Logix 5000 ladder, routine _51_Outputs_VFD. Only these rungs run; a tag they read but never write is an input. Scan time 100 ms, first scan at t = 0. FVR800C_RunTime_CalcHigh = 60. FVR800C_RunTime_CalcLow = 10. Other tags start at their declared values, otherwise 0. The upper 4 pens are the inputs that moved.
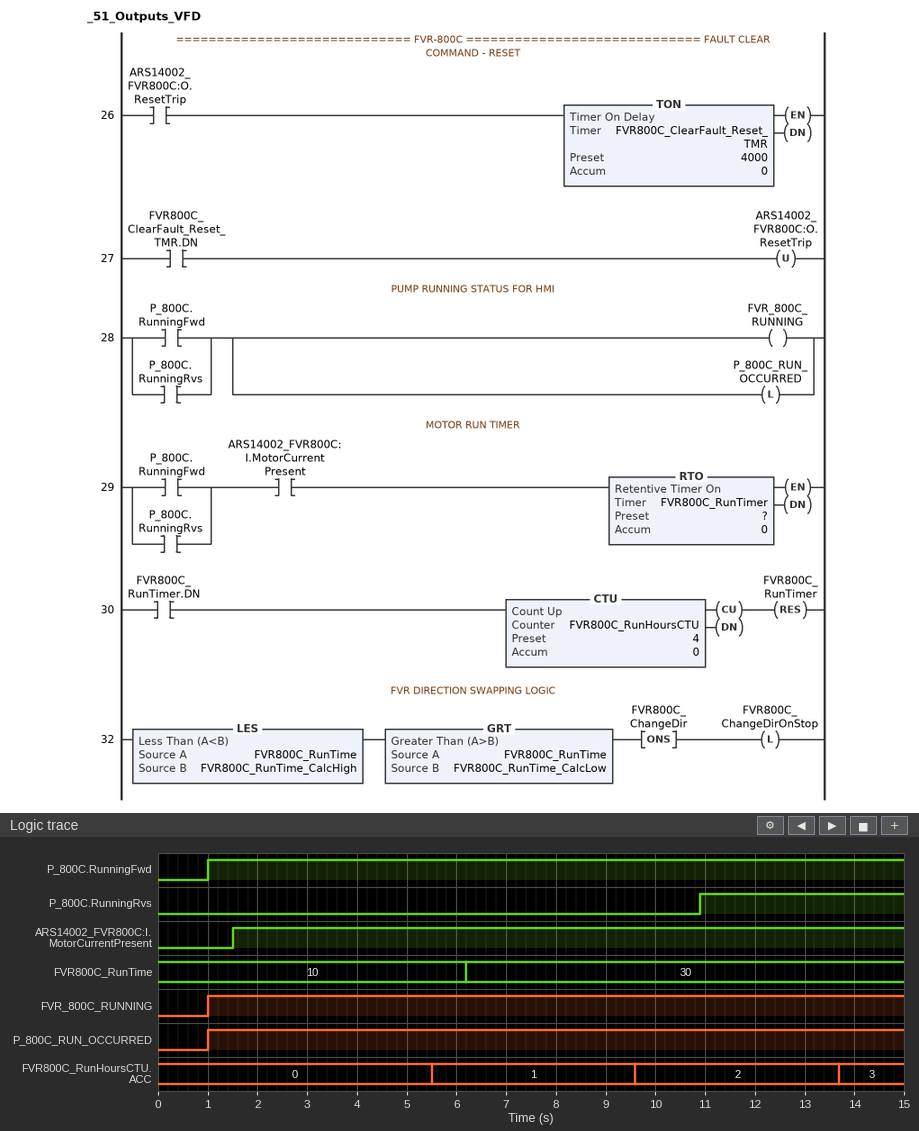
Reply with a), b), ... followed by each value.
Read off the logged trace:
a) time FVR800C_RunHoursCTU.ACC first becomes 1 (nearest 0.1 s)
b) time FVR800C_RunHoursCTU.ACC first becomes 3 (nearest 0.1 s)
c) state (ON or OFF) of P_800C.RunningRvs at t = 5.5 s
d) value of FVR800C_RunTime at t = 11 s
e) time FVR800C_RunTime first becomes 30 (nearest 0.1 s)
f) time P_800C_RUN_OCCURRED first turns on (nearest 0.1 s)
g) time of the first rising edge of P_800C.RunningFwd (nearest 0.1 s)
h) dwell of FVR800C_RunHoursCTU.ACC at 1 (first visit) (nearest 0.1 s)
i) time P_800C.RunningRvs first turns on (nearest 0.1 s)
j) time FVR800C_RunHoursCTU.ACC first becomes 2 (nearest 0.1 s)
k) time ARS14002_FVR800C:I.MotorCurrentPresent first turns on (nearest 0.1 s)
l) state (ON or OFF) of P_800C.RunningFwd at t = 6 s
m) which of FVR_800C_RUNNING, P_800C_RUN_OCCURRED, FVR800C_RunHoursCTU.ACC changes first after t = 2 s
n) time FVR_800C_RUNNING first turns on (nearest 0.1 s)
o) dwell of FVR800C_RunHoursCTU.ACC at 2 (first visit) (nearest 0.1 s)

a) 5.5 s
b) 13.7 s
c) OFF
d) 30
e) 6.2 s
f) 1.0 s
g) 1.0 s
h) 4.1 s
i) 10.9 s
j) 9.6 s
k) 1.5 s
l) ON
m) FVR800C_RunHoursCTU.ACC
n) 1.0 s
o) 4.1 s
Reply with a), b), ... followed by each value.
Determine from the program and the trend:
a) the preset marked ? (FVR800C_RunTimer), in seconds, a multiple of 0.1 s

a) 4.0 s
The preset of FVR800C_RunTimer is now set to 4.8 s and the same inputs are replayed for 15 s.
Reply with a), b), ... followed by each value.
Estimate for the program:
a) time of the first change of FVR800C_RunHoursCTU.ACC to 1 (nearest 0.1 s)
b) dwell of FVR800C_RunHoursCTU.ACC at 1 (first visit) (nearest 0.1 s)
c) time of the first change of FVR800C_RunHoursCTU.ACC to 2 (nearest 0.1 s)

a) 6.3 s
b) 4.9 s
c) 11.2 s
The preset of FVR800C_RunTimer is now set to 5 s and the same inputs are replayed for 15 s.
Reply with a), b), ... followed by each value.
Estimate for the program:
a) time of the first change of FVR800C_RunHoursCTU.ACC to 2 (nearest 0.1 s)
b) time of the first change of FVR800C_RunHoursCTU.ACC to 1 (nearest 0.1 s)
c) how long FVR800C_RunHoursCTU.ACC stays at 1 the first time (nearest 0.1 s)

a) 11.6 s
b) 6.5 s
c) 5.1 s
